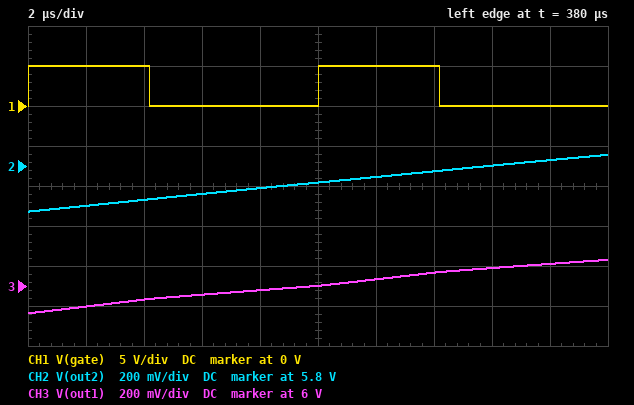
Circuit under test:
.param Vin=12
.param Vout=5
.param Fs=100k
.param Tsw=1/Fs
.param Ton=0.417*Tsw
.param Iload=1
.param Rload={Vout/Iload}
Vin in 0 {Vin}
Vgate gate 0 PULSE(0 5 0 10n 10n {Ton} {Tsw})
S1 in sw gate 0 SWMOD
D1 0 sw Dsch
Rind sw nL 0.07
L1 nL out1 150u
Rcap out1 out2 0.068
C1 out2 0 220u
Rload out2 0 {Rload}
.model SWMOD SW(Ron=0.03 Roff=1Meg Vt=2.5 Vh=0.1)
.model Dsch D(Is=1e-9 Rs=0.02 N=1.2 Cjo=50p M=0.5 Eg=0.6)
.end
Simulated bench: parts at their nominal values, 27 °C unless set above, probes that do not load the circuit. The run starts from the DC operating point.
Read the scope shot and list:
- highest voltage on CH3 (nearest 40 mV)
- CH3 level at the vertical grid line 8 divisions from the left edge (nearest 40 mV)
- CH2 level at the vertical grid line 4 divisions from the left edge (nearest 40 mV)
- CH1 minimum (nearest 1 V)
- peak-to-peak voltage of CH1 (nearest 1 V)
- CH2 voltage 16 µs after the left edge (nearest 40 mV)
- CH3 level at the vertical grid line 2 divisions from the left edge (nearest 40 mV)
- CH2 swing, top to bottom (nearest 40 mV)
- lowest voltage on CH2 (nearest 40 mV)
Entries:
6.12 V
6.08 V
5.68 V
0 V
5 V
5.80 V
5.92 V
280 mV
5.56 V
